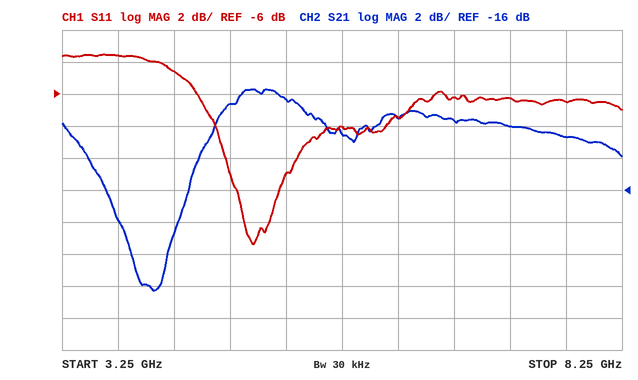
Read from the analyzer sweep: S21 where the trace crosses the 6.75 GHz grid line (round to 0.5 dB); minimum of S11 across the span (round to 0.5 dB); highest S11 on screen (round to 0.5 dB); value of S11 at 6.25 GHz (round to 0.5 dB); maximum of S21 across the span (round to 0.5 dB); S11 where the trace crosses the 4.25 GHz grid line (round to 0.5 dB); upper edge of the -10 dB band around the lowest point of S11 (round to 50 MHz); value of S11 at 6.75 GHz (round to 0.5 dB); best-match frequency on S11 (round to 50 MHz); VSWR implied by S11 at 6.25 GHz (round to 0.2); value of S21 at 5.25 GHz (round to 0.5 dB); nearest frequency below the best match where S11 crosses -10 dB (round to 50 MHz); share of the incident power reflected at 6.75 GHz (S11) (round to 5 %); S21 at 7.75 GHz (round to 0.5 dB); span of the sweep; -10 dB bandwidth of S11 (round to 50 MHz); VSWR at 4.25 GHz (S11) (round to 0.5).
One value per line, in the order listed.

-11.5 dB
-15.5 dB
-3.5 dB
-7.5 dB
-9.5 dB
-4.5 dB
5.35 GHz
-6.0 dB
4.95 GHz
2.4
-10.5 dB
4.70 GHz
25 %
-12.5 dB
5 GHz
650 MHz
4.0
